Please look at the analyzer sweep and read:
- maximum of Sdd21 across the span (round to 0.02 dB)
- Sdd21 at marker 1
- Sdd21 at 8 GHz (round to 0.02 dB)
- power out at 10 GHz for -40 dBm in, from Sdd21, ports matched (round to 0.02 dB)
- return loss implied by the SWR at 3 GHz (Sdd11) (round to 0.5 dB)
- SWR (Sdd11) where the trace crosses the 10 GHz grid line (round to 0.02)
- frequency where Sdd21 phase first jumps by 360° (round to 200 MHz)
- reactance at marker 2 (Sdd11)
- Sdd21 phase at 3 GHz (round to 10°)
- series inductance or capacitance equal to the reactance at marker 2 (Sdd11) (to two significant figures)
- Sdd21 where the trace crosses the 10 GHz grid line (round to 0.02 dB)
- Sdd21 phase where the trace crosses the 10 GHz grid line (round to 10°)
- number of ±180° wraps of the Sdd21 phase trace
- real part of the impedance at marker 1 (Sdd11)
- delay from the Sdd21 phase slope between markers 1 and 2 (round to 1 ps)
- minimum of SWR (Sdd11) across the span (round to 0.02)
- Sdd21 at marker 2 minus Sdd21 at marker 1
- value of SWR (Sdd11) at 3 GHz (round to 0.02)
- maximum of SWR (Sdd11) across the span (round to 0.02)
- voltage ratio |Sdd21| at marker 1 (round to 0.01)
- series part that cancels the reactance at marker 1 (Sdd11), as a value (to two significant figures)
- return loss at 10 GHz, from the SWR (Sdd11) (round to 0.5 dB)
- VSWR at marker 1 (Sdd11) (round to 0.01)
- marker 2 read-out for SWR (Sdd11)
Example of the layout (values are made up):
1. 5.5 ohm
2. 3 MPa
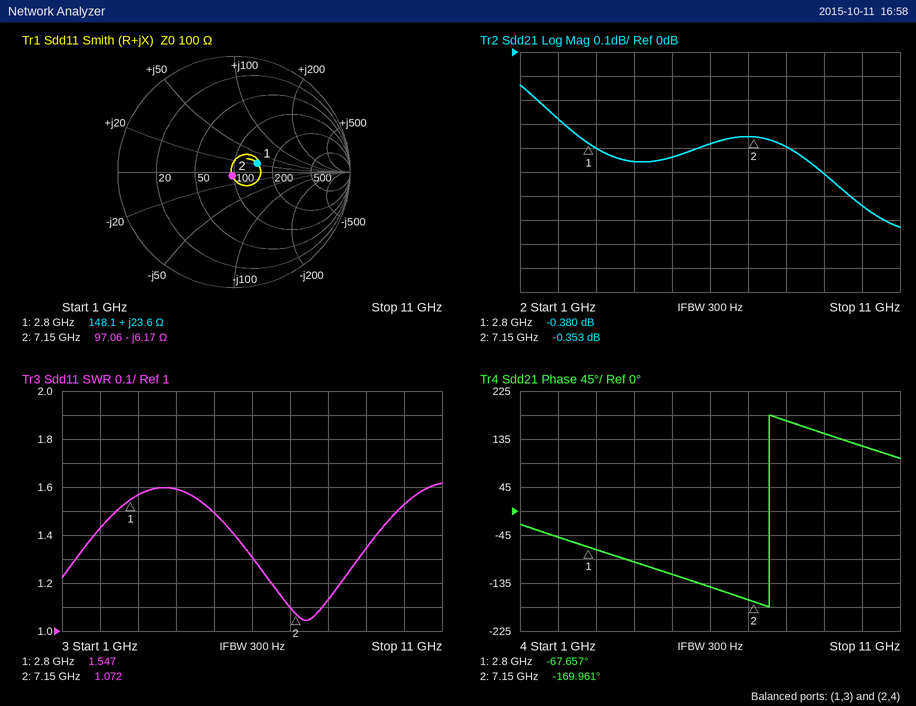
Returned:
1. -0.14 dB
2. -0.380 dB
3. -0.40 dB
4. -40.64 dBm
5. 13.0 dB
6. 1.52
7. 7.6 GHz
8. -6.17 Ω
9. -70°
10. 3.6 pF
11. -0.64 dB
12. 120°
13. 1
14. 148.1 Ω
15. 65 ps
16. 1.04
17. 0.027 dB
18. 1.56
19. 1.62
20. 0.96
21. 2.4 pF
22. 13.5 dB
23. 1.55
24. 1.072
